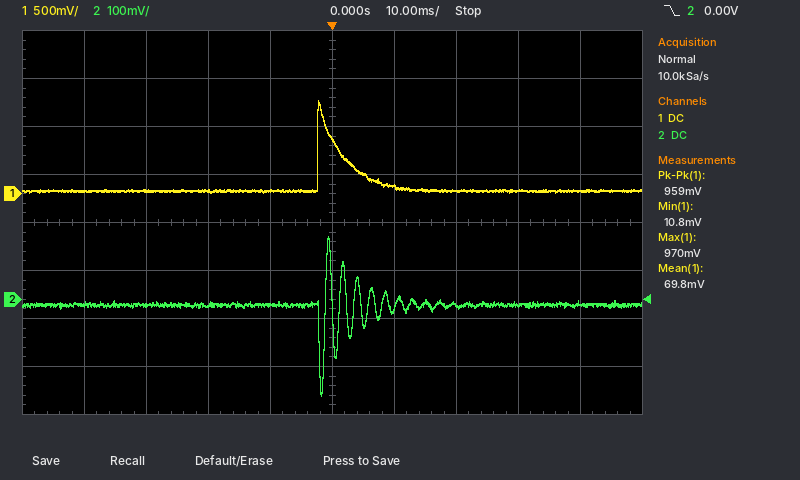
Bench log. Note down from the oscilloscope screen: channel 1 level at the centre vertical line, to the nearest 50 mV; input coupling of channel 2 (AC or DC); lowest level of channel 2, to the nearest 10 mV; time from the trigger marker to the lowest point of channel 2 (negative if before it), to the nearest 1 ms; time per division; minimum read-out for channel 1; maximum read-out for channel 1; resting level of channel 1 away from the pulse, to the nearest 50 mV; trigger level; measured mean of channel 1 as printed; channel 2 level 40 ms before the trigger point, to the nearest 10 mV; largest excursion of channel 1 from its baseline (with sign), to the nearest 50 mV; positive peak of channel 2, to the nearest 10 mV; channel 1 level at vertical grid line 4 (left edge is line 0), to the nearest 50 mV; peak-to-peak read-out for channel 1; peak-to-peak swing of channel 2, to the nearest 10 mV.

550 mV
DC
-200 mV
-2 ms
10 ms
10.8 mV
970 mV
50 mV
0.00 V
69.8 mV
-10 mV
+950 mV
130 mV
50 mV
959 mV
330 mV
